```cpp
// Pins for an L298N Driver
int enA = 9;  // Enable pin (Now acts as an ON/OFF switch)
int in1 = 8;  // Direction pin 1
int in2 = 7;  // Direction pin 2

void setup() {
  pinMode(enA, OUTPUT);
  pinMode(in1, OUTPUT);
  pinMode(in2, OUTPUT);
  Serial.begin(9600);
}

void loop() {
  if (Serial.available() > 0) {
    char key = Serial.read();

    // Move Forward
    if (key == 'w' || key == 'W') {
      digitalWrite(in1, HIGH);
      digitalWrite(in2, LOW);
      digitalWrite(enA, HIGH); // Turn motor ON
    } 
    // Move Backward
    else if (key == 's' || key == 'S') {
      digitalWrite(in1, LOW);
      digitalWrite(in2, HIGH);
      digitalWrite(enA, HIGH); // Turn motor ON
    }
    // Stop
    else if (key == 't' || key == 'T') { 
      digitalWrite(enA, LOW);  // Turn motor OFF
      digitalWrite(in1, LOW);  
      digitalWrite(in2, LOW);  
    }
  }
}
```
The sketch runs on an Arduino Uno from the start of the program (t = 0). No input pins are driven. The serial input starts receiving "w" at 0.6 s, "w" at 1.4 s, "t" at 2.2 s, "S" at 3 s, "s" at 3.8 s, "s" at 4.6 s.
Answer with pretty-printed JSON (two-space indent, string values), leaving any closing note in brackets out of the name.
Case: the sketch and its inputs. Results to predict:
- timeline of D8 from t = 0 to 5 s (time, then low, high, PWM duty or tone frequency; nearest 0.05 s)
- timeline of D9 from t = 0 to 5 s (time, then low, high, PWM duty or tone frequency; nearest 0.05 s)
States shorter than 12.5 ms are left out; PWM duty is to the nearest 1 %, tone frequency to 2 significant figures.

{
  "timeline of D8 from t = 0 to 5 s": "0 s low; 0.6 s high; 2.2 s low",
  "timeline of D9 from t = 0 to 5 s": "0 s low; 0.6 s high; 2.2 s low; 3 s high"
}
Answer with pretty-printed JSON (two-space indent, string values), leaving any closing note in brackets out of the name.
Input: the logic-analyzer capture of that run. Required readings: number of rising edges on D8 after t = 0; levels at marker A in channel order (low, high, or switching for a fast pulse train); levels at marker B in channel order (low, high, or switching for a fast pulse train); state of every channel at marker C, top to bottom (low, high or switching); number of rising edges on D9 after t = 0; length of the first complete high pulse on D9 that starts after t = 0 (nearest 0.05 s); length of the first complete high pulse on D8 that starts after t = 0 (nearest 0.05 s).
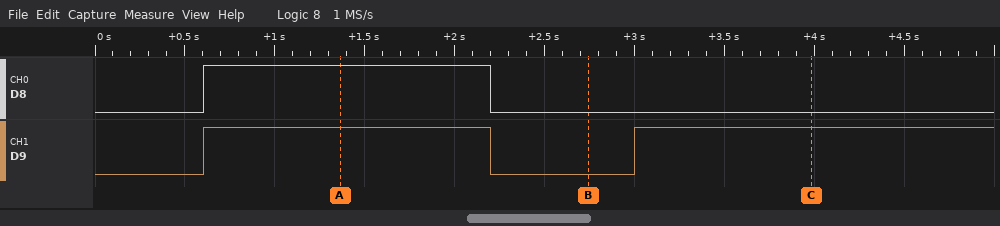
{
  "number of rising edges on D8 after t = 0": "1",
  "levels at marker A in channel order": "D8 high, D9 high",
  "levels at marker B in channel order": "D8 low, D9 low",
  "state of every channel at marker C, top to bottom": "D8 low, D9 high",
  "number of rising edges on D9 after t = 0": "2",
  "length of the first complete high pulse on D9 that starts after t = 0": "1.60 s",
  "length of the first complete high pulse on D8 that starts after t = 0": "1.60 s"
}
